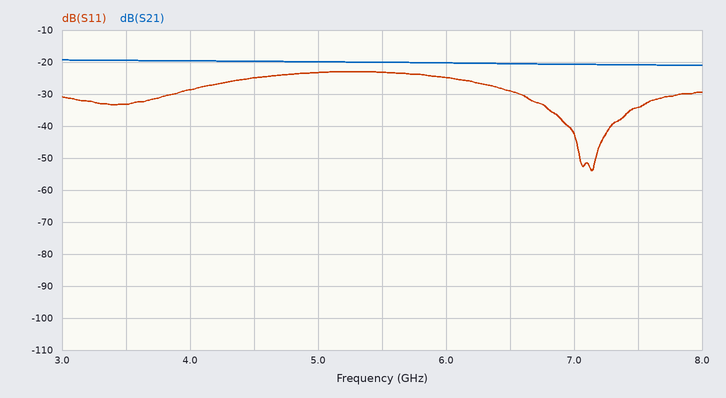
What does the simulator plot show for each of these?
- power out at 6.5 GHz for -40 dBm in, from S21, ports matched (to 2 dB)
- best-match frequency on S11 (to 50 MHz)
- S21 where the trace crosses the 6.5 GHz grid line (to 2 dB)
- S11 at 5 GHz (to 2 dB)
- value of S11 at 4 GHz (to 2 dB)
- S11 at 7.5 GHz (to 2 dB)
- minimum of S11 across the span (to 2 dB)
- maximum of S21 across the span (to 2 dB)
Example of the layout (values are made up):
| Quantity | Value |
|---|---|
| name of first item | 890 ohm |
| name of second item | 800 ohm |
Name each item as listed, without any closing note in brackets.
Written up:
| Quantity | Value |
|---|---|
| power out at 6.5 GHz for -40 dBm in, from S21, ports matched | -60 dBm |
| best-match frequency on S11 | 7.15 GHz |
| S21 where the trace crosses the 6.5 GHz grid line | -20 dB |
| S11 at 5 GHz | -24 dB |
| value of S11 at 4 GHz | -28 dB |
| S11 at 7.5 GHz | -34 dB |
| minimum of S11 across the span | -54 dB |
| maximum of S21 across the span | -20 dB |
